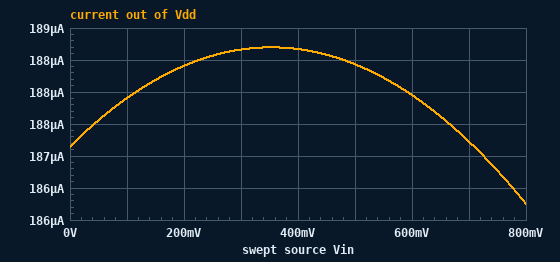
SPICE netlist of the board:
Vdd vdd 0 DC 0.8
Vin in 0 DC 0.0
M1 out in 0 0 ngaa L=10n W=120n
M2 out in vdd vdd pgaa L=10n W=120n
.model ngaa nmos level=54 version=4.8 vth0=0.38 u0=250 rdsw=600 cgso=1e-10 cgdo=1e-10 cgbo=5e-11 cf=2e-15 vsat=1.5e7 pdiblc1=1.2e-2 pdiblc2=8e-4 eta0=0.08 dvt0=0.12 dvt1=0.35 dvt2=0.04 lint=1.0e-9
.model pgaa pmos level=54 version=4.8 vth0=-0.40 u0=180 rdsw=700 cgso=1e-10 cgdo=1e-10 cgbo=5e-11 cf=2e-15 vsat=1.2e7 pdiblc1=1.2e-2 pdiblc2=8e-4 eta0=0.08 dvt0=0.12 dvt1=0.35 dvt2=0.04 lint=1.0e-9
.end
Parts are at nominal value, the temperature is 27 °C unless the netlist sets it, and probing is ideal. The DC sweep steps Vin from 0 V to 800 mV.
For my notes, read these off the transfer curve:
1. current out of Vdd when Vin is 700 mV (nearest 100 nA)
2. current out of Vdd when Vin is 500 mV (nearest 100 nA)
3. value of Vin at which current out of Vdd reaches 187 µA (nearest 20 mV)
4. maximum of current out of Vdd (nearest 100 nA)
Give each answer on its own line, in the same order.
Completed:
187.2 µA
188.4 µA
720 mV
188.7 µA
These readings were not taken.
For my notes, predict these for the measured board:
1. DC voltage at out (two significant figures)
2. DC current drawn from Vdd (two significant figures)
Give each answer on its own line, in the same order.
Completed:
410 mV
190 µA
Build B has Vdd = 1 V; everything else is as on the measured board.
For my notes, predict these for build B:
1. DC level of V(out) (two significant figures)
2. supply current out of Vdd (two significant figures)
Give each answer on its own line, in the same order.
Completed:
520 mV
270 µA
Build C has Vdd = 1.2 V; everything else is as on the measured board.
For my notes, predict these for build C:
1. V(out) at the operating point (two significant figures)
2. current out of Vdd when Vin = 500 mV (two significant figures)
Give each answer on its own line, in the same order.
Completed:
630 mV
360 µA
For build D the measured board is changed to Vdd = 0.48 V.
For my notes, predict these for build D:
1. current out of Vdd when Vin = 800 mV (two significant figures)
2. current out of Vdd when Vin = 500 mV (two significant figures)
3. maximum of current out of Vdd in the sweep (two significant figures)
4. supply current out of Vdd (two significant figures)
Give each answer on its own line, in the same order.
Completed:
80 µA
85 µA
87 µA
86 µA
